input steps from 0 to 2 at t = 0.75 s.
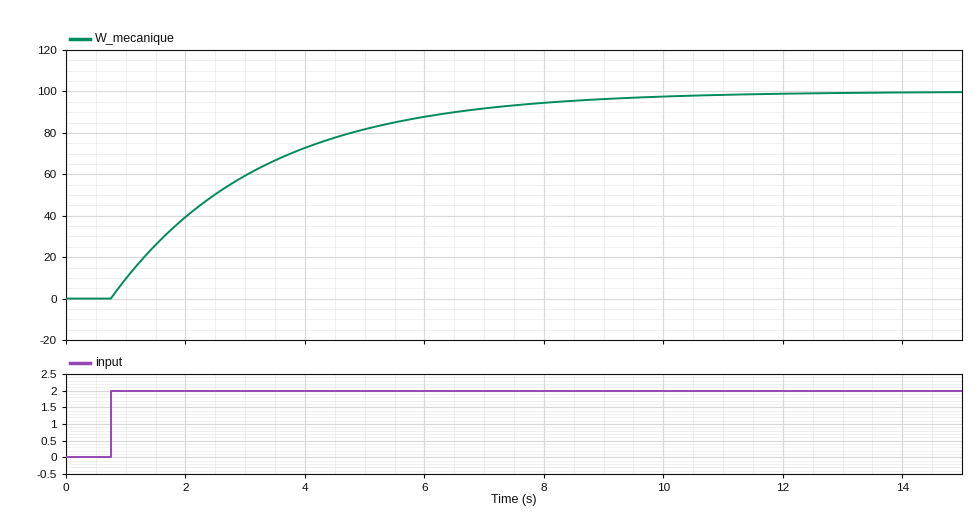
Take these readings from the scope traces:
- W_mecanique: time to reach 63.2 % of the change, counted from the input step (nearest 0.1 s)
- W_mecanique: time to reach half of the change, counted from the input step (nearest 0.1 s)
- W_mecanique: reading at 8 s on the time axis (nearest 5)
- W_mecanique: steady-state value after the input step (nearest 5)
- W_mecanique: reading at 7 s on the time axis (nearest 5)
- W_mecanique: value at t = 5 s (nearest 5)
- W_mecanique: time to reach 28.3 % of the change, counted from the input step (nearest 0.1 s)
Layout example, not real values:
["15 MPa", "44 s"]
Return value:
["2.5 s", "1.7 s", "95", "100", "90", "80", "0.8 s"]
